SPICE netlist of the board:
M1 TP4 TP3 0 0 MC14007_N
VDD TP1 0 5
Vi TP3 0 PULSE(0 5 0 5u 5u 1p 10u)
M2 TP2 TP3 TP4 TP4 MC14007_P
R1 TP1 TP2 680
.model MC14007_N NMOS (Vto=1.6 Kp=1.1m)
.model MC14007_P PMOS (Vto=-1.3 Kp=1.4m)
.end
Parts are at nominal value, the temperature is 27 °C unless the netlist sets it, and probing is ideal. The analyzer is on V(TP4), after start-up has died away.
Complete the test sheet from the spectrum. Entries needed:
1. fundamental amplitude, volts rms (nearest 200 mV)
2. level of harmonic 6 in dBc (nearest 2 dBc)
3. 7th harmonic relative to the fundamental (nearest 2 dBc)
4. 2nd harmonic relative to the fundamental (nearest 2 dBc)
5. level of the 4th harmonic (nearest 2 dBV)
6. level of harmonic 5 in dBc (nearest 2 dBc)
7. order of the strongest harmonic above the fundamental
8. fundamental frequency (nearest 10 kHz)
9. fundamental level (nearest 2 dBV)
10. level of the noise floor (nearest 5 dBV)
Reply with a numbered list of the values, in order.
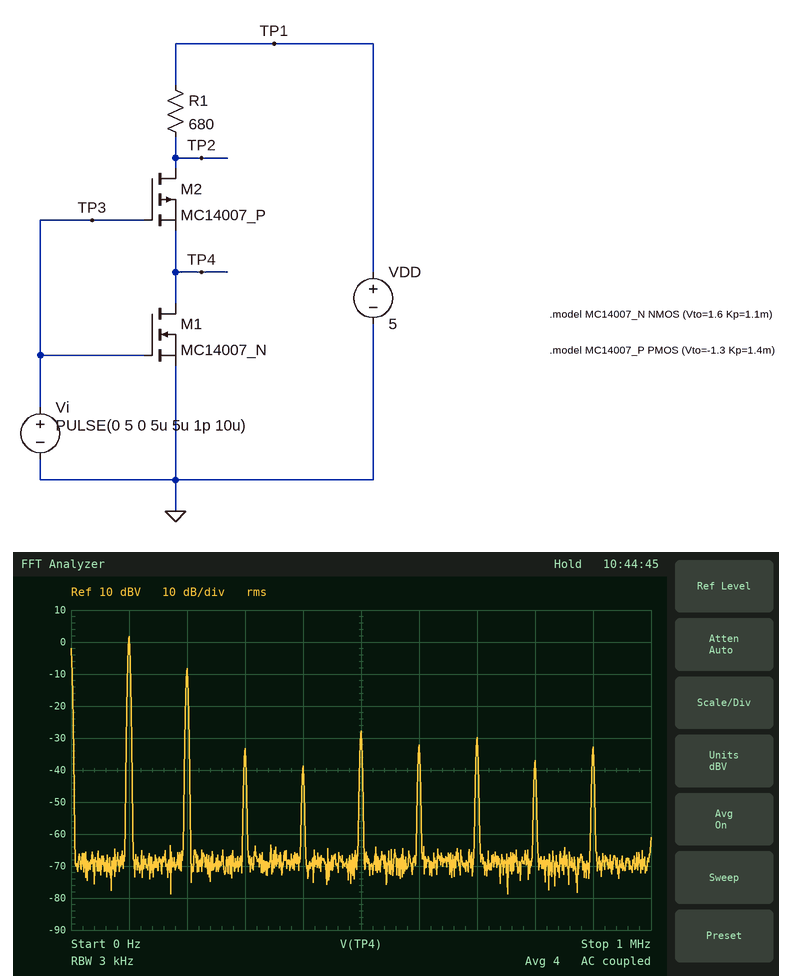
1. 1.2 V
2. -34 dBc
3. -32 dBc
4. -10 dBc
5. -38 dBV
6. -30 dBc
7. 2
8. 100 kHz
9. 2 dBV
10. -70 dBV
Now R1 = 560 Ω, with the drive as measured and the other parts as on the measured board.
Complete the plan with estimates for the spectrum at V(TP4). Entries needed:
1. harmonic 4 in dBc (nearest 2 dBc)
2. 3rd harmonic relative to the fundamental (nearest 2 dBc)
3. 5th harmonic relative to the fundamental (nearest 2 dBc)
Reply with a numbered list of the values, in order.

1. -30 dBc
2. -60 dBc
3. -26 dBc
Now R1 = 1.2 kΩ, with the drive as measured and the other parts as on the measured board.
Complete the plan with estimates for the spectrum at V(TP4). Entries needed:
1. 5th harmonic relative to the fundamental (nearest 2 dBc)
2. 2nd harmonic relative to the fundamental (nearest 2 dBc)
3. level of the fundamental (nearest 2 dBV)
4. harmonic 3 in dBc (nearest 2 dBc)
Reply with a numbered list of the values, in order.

1. -36 dBc
2. -12 dBc
3. 4 dBV
4. -20 dBc
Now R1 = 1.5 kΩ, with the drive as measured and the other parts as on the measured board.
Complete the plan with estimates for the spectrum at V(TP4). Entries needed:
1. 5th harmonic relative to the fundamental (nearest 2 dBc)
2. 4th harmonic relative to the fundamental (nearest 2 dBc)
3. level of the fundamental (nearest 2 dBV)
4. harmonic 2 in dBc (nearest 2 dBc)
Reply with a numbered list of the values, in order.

1. -32 dBc
2. -26 dBc
3. 4 dBV
4. -14 dBc
